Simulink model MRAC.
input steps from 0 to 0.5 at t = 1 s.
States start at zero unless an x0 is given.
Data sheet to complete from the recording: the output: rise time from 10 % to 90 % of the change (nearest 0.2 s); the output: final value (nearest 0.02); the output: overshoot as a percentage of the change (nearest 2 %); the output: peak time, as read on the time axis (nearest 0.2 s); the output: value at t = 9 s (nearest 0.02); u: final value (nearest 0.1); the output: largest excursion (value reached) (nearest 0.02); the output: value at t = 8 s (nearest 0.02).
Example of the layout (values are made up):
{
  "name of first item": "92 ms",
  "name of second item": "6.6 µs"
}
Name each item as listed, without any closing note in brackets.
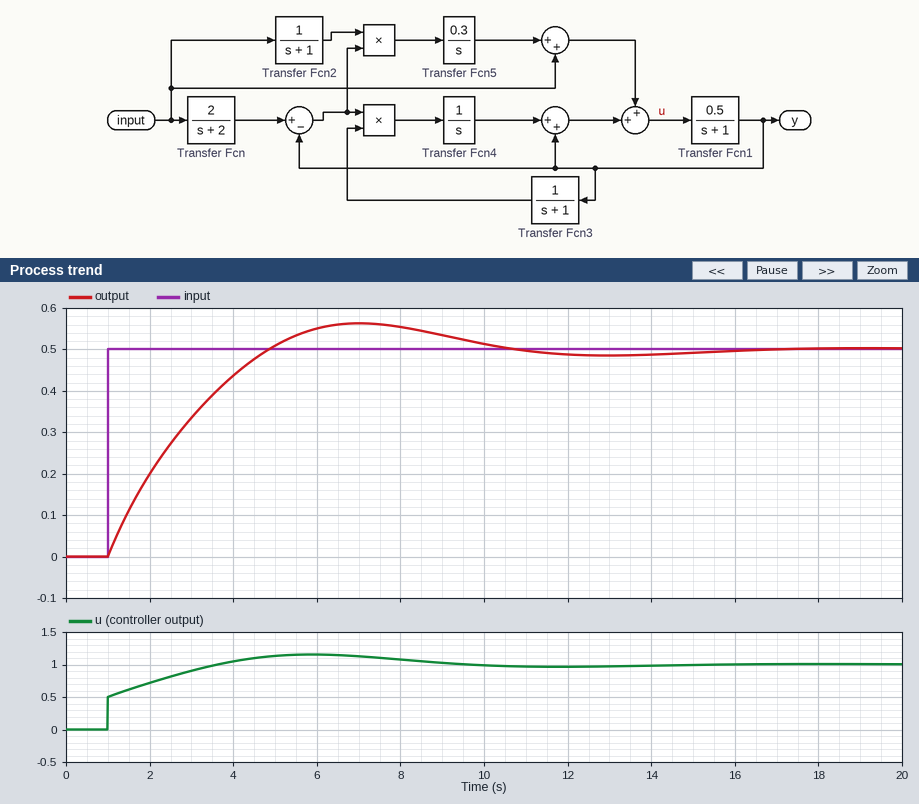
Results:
{
  "the output: rise time from 10 % to 90 % of the change": "3.0 s",
  "the output: final value": "0.50",
  "the output: overshoot as a percentage of the change": "12 %",
  "the output: peak time, as read on the time axis": "7.0 s",
  "the output: value at t = 9 s": "0.54",
  "u: final value": "1.0",
  "the output: largest excursion (value reached)": "0.56",
  "the output: value at t = 8 s": "0.56"
}
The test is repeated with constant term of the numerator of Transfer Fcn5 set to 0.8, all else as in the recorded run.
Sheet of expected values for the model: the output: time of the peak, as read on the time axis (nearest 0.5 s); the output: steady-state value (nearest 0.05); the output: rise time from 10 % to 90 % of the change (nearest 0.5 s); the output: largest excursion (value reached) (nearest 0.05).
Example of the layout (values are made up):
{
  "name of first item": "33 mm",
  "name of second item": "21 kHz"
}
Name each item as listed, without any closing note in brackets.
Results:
{
  "the output: time of the peak, as read on the time axis": "6.0 s",
  "the output: steady-state value": "0.50",
  "the output: rise time from 10 % to 90 % of the change": "2.5 s",
  "the output: largest excursion (value reached)": "0.60"
}
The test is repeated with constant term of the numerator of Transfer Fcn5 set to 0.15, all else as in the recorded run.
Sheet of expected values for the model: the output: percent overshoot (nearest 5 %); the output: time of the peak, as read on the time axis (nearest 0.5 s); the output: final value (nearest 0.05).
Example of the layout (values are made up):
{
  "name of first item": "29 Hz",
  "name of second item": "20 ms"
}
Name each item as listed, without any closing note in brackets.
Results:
{
  "the output: percent overshoot": "10 %",
  "the output: time of the peak, as read on the time axis": "7.5 s",
  "the output: final value": "0.50"
}
